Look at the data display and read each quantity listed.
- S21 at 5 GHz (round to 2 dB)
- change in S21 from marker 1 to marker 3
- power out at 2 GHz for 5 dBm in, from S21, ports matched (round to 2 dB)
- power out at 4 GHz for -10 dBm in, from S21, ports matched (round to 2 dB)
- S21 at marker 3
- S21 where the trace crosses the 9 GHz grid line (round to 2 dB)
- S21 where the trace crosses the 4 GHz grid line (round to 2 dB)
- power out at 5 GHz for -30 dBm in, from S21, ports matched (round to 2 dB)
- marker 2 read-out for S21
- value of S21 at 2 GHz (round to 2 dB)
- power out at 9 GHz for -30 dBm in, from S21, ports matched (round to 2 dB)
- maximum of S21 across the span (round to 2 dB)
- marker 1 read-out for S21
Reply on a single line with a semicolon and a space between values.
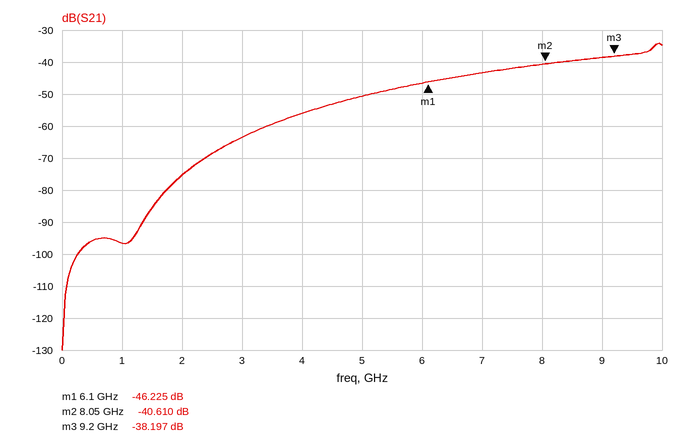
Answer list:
-50 dB; 8.028 dB; -70 dBm; -66 dBm; -38.197 dB; -38 dB; -56 dB; -80 dBm; -40.610 dB; -76 dB; -68 dBm; -34 dB; -46.225 dB
